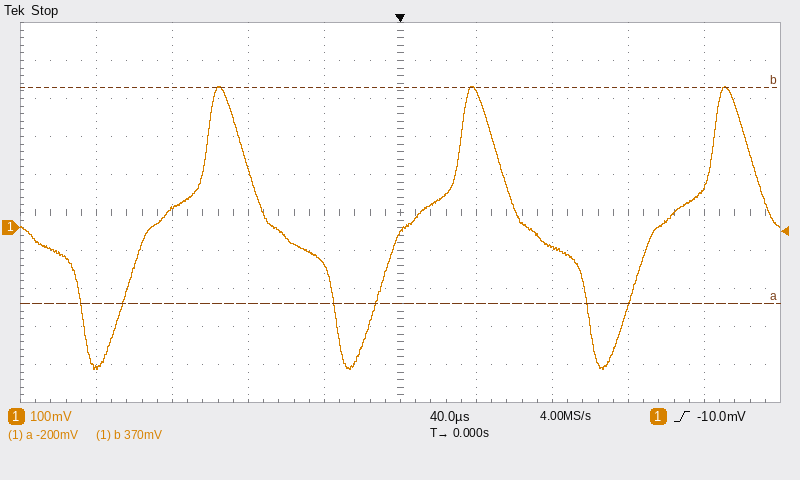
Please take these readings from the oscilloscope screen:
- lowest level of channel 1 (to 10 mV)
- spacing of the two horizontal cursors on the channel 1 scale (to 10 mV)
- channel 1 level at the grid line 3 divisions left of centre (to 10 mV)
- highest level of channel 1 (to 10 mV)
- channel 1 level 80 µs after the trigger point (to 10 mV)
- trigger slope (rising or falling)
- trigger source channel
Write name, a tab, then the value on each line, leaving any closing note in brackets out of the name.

lowest level of channel 1	-370 mV
spacing of the two horizontal cursors on the channel 1 scale	570 mV
channel 1 level at the grid line 3 divisions left of centre	50 mV
highest level of channel 1	370 mV
channel 1 level 80 µs after the trigger point	-50 mV
trigger slope	rising
trigger source channel	channel 1
